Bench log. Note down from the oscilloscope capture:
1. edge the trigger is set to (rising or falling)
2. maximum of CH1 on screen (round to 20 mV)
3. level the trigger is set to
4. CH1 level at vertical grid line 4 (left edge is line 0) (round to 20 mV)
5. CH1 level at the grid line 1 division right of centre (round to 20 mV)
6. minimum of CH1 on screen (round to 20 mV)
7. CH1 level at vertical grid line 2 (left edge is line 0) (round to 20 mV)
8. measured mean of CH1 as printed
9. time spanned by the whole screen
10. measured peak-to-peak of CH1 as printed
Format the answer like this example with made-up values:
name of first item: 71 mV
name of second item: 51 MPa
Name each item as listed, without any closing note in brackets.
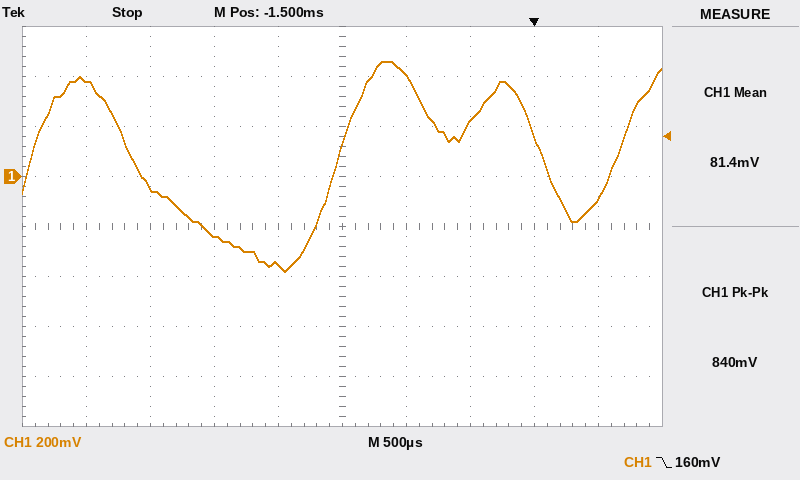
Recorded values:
edge the trigger is set to: falling
maximum of CH1 on screen: 460 mV
level the trigger is set to: 160 mV
CH1 level at vertical grid line 4 (left edge is line 0): -360 mV
CH1 level at the grid line 1 division right of centre: 400 mV
minimum of CH1 on screen: -380 mV
CH1 level at vertical grid line 2 (left edge is line 0): -40 mV
measured mean of CH1 as printed: 81.4 mV
time spanned by the whole screen: 5 ms
measured peak-to-peak of CH1 as printed: 840 mV
